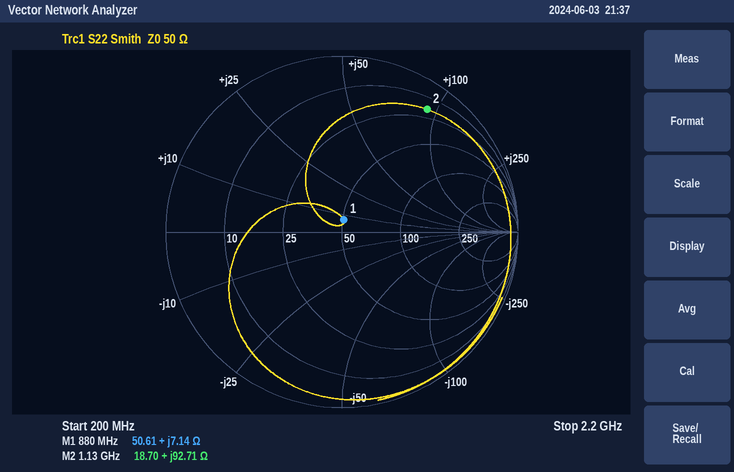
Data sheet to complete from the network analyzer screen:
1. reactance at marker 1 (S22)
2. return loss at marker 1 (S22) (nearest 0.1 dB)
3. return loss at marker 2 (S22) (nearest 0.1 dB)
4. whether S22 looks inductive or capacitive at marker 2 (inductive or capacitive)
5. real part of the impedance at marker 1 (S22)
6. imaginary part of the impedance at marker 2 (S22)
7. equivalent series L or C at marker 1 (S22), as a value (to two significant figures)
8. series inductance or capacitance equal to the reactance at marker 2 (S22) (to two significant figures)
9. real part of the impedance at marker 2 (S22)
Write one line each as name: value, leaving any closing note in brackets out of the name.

reactance at marker 1: +7.14 Ω
return loss at marker 1 (S22): 23.0 dB
return loss at marker 2 (S22): 1.4 dB
whether S22 looks inductive or capacitive at marker 2: inductive
real part of the impedance at marker 1: 50.61 Ω
imaginary part of the impedance at marker 2: +92.71 Ω
equivalent series L or C at marker 1 (S22), as a value: 1.3 nH
series inductance or capacitance equal to the reactance at marker 2 (S22): 13 nH
real part of the impedance at marker 2: 18.70 Ω
